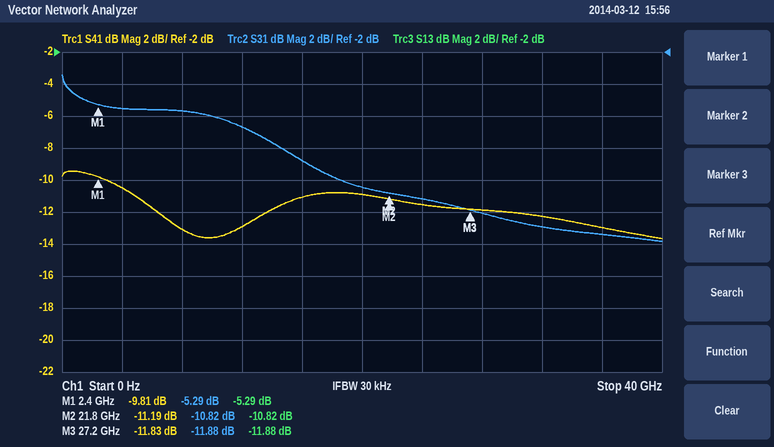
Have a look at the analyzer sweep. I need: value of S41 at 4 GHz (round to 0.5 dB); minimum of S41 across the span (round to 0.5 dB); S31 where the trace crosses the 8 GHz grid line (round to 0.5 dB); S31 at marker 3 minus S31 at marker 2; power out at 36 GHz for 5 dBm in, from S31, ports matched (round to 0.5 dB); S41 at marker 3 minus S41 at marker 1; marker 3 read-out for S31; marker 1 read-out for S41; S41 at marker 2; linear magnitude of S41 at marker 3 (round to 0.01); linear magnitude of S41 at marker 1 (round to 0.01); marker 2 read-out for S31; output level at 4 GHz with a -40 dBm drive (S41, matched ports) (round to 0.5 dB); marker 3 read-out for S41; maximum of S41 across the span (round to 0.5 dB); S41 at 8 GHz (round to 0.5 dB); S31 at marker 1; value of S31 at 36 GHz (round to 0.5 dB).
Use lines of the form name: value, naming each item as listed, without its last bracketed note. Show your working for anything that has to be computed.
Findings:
value of S41 at 4 GHz: -10.5 dB
minimum of S41 across the span: -13.5 dB
S31 where the trace crosses the 8 GHz grid line: -5.5 dB
S31 at marker 3 minus S31 at marker 2: -11.88 − (-10.82) = -1.06 dB
power out at 36 GHz for 5 dBm in, from S31, ports matched: 5 dBm + (-13.5 dB) = -8.5 dBm
S41 at marker 3 minus S41 at marker 1: -11.83 − (-9.81) = -2.02 dB
marker 3 read-out for S31: -11.88 dB
marker 1 read-out for S41: -9.81 dB
S41 at marker 2: -11.19 dB
linear magnitude of S41 at marker 3: 10^(-11.83/20) ≈ 0.26
linear magnitude of S41 at marker 1: 10^(-9.81/20) ≈ 0.32
marker 2 read-out for S31: -10.82 dB
output level at 4 GHz with a -40 dBm drive (S41, matched ports): -40 dBm + (-10.5 dB) = -50.5 dBm
marker 3 read-out for S41: -11.83 dB
maximum of S41 across the span: -9.5 dB
S41 at 8 GHz: -13.0 dB
S31 at marker 1: -5.29 dB
value of S31 at 36 GHz: -13.5 dB
